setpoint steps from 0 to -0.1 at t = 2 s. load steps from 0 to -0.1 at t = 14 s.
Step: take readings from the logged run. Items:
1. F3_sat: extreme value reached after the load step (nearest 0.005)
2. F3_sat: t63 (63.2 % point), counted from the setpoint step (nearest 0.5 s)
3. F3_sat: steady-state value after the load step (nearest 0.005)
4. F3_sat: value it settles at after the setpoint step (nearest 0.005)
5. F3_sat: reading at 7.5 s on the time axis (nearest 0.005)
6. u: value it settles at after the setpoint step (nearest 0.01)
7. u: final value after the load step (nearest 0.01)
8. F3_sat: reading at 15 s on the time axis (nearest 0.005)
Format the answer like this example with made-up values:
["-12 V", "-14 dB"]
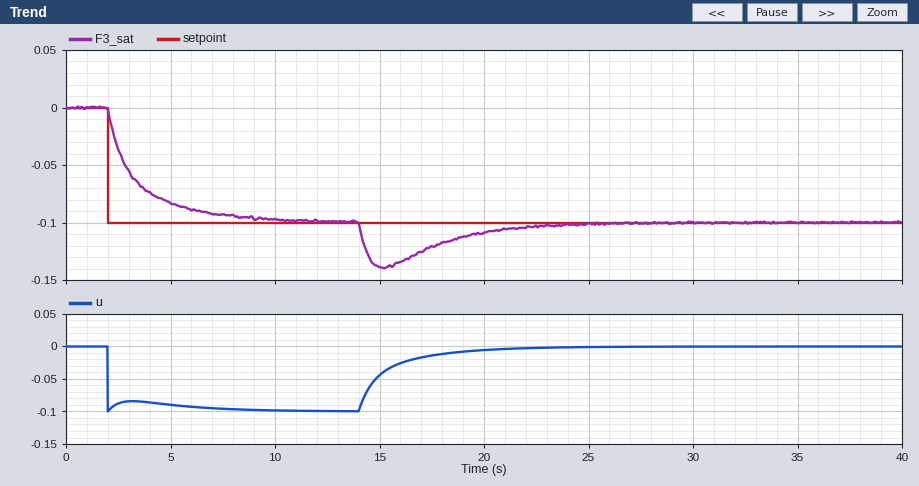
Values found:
["-0.140", "1.5 s", "-0.100", "-0.100", "-0.095", "-0.10", "0.00", "-0.140"]
